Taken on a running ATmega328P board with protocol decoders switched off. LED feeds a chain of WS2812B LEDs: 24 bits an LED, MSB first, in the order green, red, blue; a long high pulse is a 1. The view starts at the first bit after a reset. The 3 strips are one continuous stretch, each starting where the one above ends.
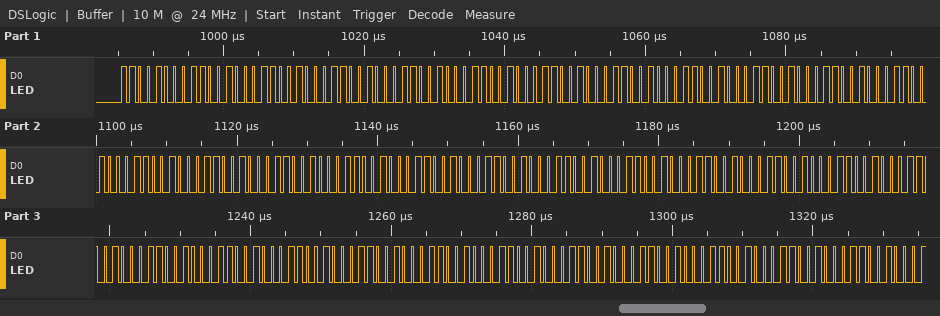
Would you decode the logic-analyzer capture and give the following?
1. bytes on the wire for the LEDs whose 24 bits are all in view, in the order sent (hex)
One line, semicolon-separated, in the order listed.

C8 C8 C8 C8 C8 C8 C8 C8 C8 C8 C8 C8 C8 C8 C8 C8 C8 C8 C8 C8 C8 C8 C8 C8 C8 C8 C8 C8 C8 C8 C8 C8 C8
